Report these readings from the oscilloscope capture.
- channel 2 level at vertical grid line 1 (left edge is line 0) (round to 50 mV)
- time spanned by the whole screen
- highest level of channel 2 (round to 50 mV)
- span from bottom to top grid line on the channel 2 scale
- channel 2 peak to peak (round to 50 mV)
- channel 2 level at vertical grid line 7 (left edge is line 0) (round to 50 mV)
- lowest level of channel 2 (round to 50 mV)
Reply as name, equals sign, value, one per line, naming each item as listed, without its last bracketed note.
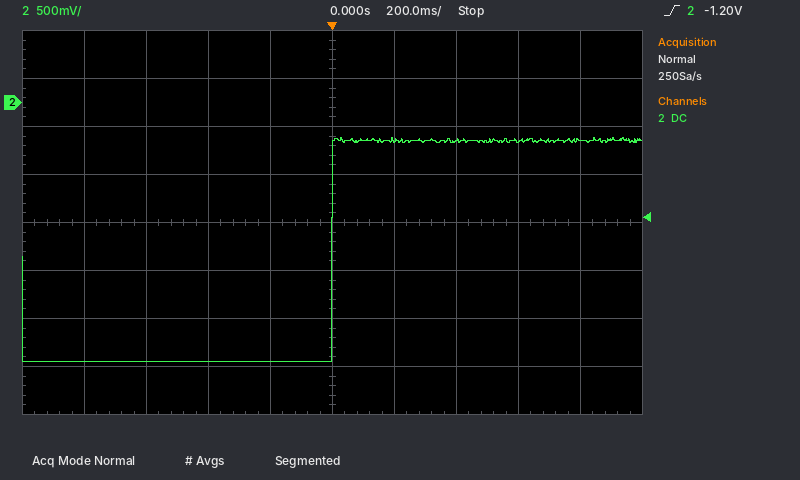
channel 2 level at vertical grid line 1 (left edge is line 0) = -2.70 V
time spanned by the whole screen = 2 s
highest level of channel 2 = -350 mV
span from bottom to top grid line on the channel 2 scale = 4 V
channel 2 peak to peak = 2.35 V
channel 2 level at vertical grid line 7 (left edge is line 0) = -400 mV
lowest level of channel 2 = -2.70 V
